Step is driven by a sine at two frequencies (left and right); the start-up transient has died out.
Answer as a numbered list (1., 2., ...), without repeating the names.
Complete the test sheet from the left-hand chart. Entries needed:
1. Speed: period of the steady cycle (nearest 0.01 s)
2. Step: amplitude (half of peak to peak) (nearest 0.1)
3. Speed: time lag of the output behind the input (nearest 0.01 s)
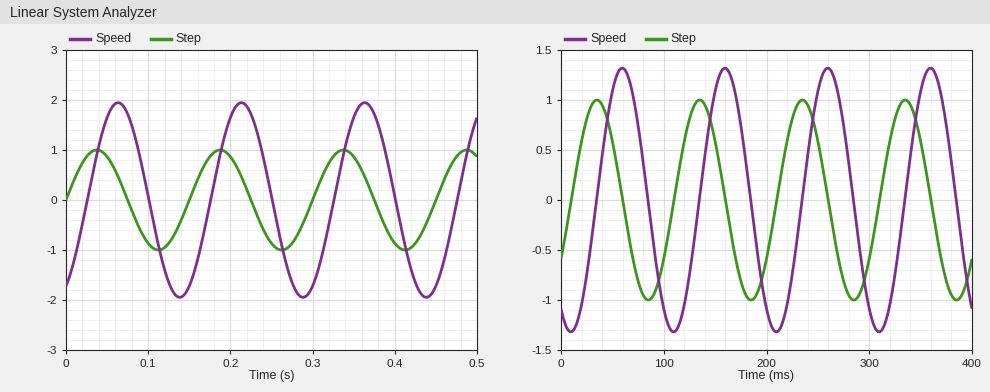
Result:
1. 0.15 s
2. 1.0
3. 0.03 s
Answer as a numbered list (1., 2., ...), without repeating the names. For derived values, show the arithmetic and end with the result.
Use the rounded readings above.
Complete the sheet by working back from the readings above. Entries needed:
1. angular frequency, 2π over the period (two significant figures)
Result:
1. 2π / 0.15 = 42 rad/s
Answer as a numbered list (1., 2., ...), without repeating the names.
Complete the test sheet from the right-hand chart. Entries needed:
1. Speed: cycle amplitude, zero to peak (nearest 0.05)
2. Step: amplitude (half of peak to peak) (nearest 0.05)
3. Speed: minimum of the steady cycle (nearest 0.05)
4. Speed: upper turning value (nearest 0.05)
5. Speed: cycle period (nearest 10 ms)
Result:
1. 1.30
2. 1.00
3. -1.30
4. 1.30
5. 100 ms
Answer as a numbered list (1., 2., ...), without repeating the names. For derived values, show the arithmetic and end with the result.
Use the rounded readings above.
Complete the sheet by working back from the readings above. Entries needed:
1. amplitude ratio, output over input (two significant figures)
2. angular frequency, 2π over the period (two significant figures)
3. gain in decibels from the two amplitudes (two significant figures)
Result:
1. 1.3 / 1 = 1.3
2. 2π / 100 = 0.063 rad/ms
3. 20 log10(1.3 / 1) = 2.3 dB
